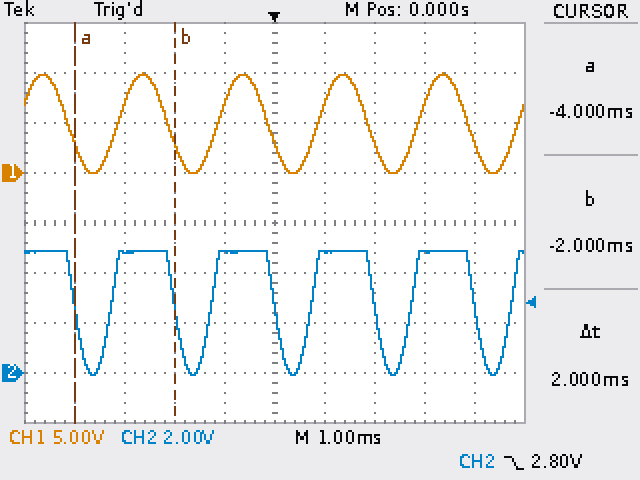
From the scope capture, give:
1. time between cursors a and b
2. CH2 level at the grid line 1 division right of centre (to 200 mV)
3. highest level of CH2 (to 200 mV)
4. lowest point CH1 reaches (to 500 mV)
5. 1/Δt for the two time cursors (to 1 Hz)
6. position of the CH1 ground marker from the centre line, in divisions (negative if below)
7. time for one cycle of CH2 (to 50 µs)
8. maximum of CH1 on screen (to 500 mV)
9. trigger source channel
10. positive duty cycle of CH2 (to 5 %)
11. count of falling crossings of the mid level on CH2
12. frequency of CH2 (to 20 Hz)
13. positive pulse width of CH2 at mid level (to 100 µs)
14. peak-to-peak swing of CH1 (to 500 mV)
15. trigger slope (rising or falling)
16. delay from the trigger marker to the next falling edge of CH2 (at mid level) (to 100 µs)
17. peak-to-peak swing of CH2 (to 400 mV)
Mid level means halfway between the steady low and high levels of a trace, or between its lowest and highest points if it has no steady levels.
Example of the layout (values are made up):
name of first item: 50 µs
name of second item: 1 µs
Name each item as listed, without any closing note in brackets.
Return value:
time between cursors a and b: 2 ms
CH2 level at the grid line 1 division right of centre: 4.8 V
highest level of CH2: 4.8 V
lowest point CH1 reaches: 0.0 V
1/Δt for the two time cursors: 500 Hz
position of the CH1 ground marker from the centre line, in divisions: +1.0 div
time for one cycle of CH2: 2.00 ms
maximum of CH1 on screen: 10.0 V
trigger source channel: CH2
positive duty cycle of CH2: 65 %
count of falling crossings of the mid level on CH2: 5
frequency of CH2: 500 Hz
positive pulse width of CH2 at mid level: 1.3 ms
peak-to-peak swing of CH1: 10.0 V
trigger slope: falling
delay from the trigger marker to the next falling edge of CH2 (at mid level): 2.0 ms
peak-to-peak swing of CH2: 4.8 V
